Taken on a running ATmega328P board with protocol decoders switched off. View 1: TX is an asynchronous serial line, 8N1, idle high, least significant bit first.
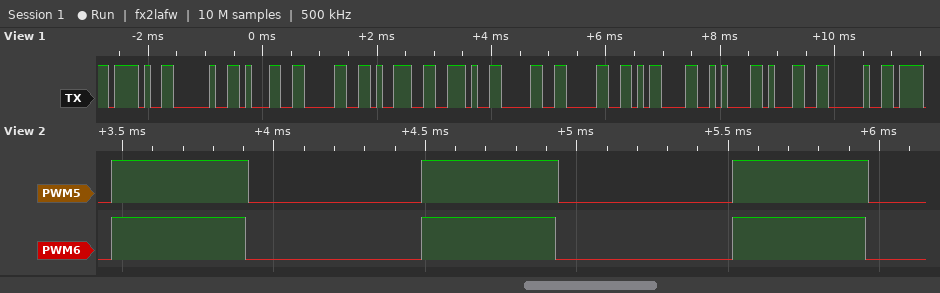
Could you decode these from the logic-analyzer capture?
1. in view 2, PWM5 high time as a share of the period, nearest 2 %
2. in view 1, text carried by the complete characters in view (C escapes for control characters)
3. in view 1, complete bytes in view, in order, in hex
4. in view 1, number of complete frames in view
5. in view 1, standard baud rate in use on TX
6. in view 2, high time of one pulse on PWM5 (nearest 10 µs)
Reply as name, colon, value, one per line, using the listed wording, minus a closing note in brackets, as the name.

in view 2, PWM5 high time as a share of the period, nearest 2 %: 44 %
in view 1, text carried by the complete characters in view: "/ 109.00\r\n1 "
in view 1, complete bytes in view, in order, in hex: 2F 20 31 30 39 2E 30 30 0D 0A 31 20
in view 1, number of complete frames in view: 12
in view 1, standard baud rate in use on TX: 9600 baud
in view 2, high time of one pulse on PWM5: 450 µs
